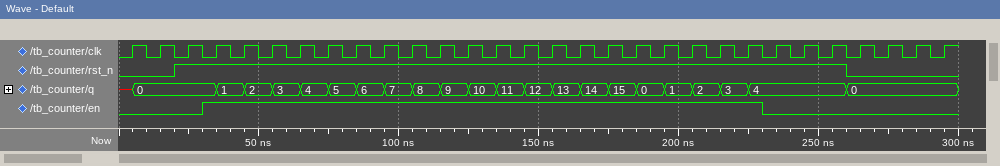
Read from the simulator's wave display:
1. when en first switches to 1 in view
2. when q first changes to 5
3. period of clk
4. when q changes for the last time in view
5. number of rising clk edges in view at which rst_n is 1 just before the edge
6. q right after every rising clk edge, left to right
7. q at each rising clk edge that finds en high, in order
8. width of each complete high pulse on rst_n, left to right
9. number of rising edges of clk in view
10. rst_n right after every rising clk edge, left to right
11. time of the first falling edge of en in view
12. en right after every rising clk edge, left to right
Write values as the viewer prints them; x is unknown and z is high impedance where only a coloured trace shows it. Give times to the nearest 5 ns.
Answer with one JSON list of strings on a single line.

["30 ns", "75 ns", "10 ns", "260 ns", "24", "0, 0, 0, 1, 2, 3, 4, 5, 6, 7, 8, 9, 10, 11, 12, 13, 14, 15, 0, 1, 2, 3, 4, 4, 4, 4, 0, 0, 0, 0", "0, 1, 2, 3, 4, 5, 6, 7, 8, 9, 10, 11, 12, 13, 14, 15, 0, 1, 2, 3", "240 ns", "30", "0 0 1 1 1 1 1 1 1 1 1 1 1 1 1 1 1 1 1 1 1 1 1 1 1 1 0 0 0 0", "230 ns", "0 0 0 1 1 1 1 1 1 1 1 1 1 1 1 1 1 1 1 1 1 1 1 0 0 0 0 0 0 0"]
